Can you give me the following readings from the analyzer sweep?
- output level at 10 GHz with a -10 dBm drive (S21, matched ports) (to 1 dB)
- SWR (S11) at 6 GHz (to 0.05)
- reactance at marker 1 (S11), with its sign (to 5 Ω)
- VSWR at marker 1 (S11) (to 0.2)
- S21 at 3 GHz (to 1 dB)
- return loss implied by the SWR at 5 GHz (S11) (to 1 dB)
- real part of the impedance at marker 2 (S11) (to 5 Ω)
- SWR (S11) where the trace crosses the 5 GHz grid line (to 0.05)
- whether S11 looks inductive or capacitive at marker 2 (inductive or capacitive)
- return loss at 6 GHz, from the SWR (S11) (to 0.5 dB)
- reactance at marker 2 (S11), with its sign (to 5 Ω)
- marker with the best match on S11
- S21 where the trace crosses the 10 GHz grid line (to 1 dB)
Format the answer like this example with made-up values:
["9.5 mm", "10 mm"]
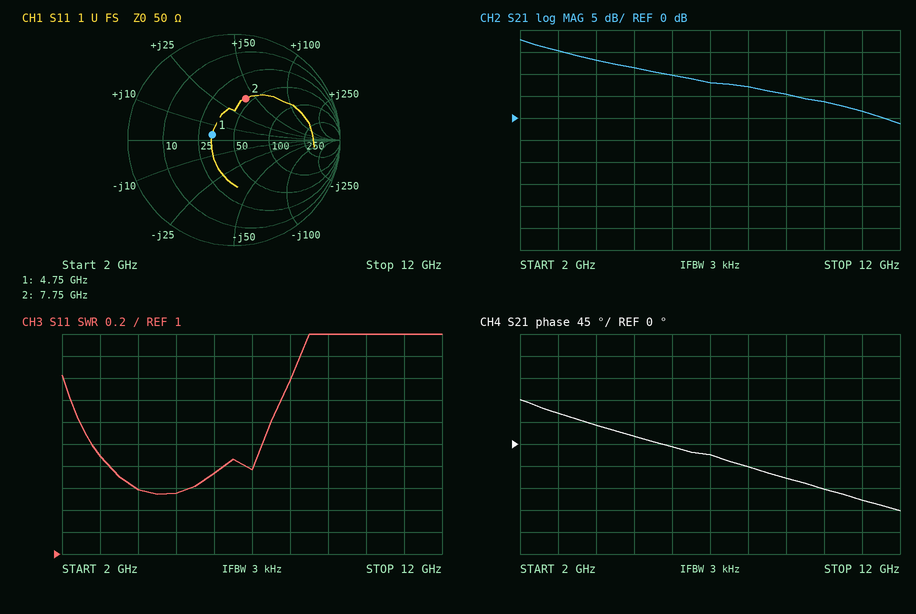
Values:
["-6 dBm", "1.75", "+5 Ω", "1.6", "15 dB", "13 dB", "45 Ω", "1.55", "inductive", "11.5 dB", "+40 Ω", "marker 1", "4 dB"]
